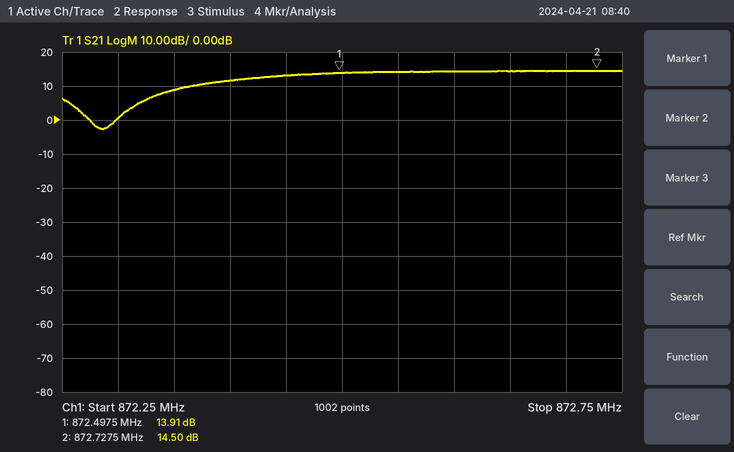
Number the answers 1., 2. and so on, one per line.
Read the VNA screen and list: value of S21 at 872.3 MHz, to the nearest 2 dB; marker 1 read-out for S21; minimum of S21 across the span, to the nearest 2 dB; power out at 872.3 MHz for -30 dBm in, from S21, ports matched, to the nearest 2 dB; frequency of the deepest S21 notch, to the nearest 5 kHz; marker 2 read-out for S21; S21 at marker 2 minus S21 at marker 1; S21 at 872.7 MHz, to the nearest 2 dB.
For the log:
1. 0 dB
2. 13.91 dB
3. -2 dB
4. -30 dBm
5. 872.285 MHz
6. 14.50 dB
7. 0.59 dB
8. 14 dB
